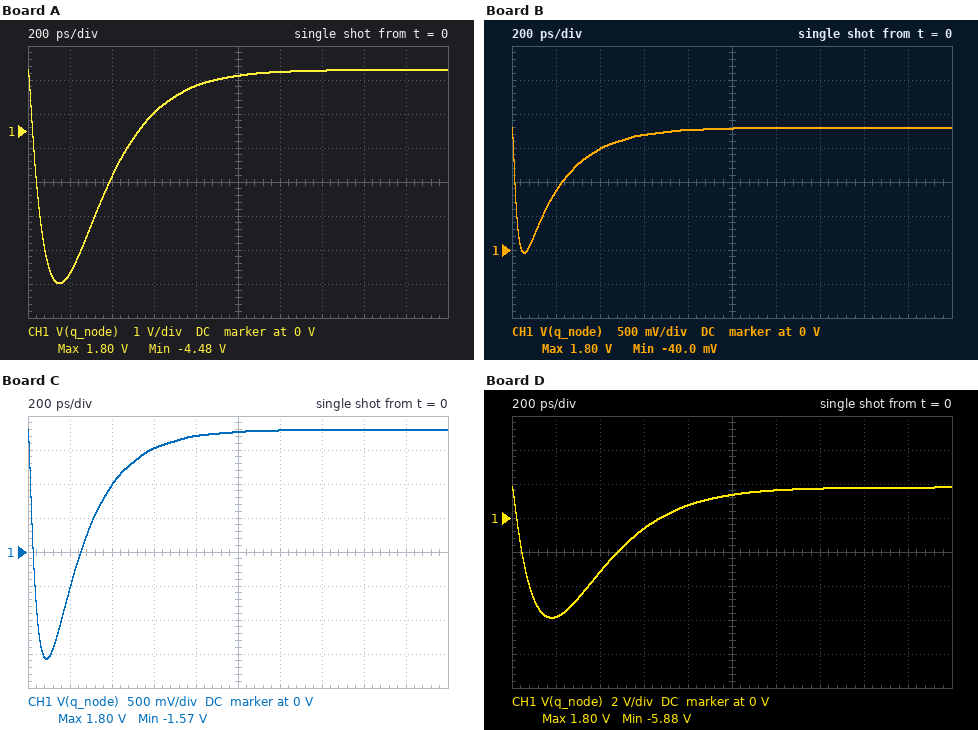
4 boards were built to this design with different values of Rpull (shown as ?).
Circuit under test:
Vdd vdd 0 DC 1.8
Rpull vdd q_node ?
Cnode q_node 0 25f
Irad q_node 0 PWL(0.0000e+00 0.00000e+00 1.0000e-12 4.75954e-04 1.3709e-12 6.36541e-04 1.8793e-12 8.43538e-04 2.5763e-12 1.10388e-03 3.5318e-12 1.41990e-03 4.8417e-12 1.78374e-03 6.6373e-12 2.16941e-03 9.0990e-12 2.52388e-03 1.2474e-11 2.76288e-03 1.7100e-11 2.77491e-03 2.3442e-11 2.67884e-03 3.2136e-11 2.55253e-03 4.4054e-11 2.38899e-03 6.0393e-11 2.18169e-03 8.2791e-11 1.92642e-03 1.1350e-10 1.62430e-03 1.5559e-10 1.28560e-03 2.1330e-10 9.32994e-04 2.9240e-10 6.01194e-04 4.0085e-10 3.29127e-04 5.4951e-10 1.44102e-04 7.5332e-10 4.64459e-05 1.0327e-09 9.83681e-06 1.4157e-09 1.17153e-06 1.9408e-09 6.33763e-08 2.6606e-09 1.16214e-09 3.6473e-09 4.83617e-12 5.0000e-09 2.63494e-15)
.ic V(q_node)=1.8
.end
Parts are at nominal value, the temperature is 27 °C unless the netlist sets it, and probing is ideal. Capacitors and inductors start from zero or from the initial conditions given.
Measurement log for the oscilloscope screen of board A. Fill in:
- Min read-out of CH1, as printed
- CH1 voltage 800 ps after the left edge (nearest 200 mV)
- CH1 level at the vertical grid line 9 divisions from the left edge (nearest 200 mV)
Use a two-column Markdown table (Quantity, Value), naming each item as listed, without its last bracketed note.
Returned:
| Quantity | Value |
|---|---|
| Min read-out of CH1, as printed | -4.48 V |
| CH1 voltage 800 ps after the left edge | 1.4 V |
| CH1 level at the vertical grid line 9 divisions from the left edge | 1.8 V |
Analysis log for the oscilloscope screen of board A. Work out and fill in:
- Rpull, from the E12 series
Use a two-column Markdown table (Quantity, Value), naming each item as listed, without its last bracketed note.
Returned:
| Quantity | Value |
|---|---|
| Rpull, from the E12 series | 4.7 kΩ |
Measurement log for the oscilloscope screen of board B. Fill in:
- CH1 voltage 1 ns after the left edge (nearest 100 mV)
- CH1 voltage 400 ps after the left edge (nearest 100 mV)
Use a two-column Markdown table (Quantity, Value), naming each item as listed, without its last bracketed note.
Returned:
| Quantity | Value |
|---|---|
| CH1 voltage 1 ns after the left edge | 1.8 V |
| CH1 voltage 400 ps after the left edge | 1.5 V |
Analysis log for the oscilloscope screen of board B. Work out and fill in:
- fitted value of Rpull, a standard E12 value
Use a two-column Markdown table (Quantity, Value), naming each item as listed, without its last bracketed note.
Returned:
| Quantity | Value |
|---|---|
| fitted value of Rpull, a standard E12 value | 820 Ω |
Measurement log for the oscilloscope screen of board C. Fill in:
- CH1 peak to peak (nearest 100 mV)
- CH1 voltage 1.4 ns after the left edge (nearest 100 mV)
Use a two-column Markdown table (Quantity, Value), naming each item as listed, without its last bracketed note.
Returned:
| Quantity | Value |
|---|---|
| CH1 peak to peak | 3.4 V |
| CH1 voltage 1.4 ns after the left edge | 1.8 V |
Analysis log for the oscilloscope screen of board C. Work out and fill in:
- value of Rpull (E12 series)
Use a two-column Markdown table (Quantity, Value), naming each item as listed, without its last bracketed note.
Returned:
| Quantity | Value |
|---|---|
| value of Rpull | 1.8 kΩ |
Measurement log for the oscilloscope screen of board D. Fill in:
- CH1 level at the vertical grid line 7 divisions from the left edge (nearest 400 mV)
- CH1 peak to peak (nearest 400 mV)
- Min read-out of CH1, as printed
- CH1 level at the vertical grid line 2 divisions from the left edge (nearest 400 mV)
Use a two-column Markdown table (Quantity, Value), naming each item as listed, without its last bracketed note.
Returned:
| Quantity | Value |
|---|---|
| CH1 level at the vertical grid line 7 divisions from the left edge | 1.6 V |
| CH1 peak to peak | 7.6 V |
| Min read-out of CH1, as printed | -5.88 V |
| CH1 level at the vertical grid line 2 divisions from the left edge | -3.2 V |
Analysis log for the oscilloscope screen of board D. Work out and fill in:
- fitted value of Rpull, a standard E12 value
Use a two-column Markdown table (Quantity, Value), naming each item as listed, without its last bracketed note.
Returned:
| Quantity | Value |
|---|---|
| fitted value of Rpull, a standard E12 value | 6.8 kΩ |
